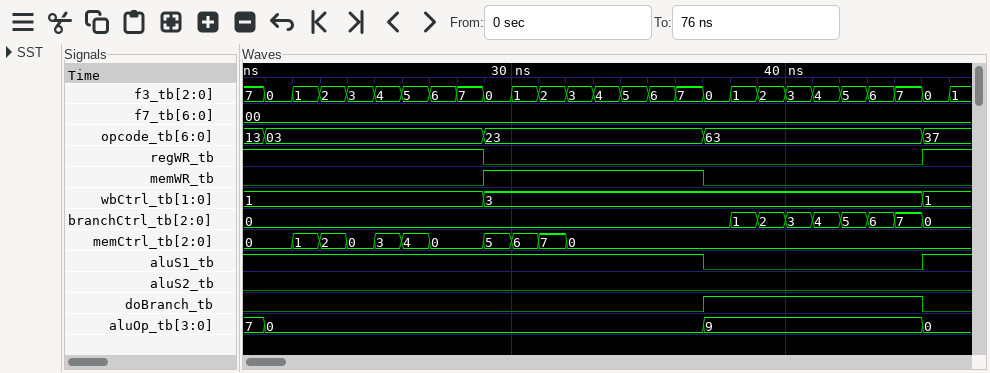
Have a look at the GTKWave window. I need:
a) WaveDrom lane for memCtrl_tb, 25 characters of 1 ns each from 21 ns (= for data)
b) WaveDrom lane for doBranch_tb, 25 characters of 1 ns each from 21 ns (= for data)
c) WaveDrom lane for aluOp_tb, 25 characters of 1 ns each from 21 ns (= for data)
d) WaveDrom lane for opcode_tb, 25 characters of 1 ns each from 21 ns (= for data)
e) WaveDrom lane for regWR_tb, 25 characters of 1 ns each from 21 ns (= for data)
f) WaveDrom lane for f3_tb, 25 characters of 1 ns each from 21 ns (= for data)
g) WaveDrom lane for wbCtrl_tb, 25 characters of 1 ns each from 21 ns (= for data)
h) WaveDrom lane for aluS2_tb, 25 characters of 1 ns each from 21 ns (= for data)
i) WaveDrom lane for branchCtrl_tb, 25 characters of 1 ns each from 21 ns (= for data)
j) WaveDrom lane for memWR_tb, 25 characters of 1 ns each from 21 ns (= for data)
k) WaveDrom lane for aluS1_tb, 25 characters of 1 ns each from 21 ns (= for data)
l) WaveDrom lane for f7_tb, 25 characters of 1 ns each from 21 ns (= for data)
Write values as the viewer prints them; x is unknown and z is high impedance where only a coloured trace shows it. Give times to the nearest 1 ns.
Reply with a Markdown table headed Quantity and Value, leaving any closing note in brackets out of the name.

| Quantity | Value |
|---|---|
| WaveDrom lane for memCtrl_tb, 25 characters of 1 ns each from 21 ns | {name: 'memCtrl_tb', wave: '=======.====.............', data: '0 1 2 0 3 4 0 5 6 7 0'} |
| WaveDrom lane for doBranch_tb, 25 characters of 1 ns each from 21 ns | {name: 'doBranch_tb', wave: '0...............1.......0'} |
| WaveDrom lane for aluOp_tb, 25 characters of 1 ns each from 21 ns | {name: 'aluOp_tb', wave: '=...............=.......=', data: '0 9 0'} |
| WaveDrom lane for opcode_tb, 25 characters of 1 ns each from 21 ns | {name: 'opcode_tb', wave: '=.......=.......=.......=', data: '03 23 63 37'} |
| WaveDrom lane for regWR_tb, 25 characters of 1 ns each from 21 ns | {name: 'regWR_tb', wave: '1.......0...............1'} |
| WaveDrom lane for f3_tb, 25 characters of 1 ns each from 21 ns | {name: 'f3_tb', wave: '=========================', data: '0 1 2 3 4 5 6 7 0 1 2 3 4 5 6 7 0 1 2 3 4 5 6 7 0'} |
| WaveDrom lane for wbCtrl_tb, 25 characters of 1 ns each from 21 ns | {name: 'wbCtrl_tb', wave: '=.......=...............=', data: '1 3 1'} |
| WaveDrom lane for aluS2_tb, 25 characters of 1 ns each from 21 ns | {name: 'aluS2_tb', wave: '0........................'} |
| WaveDrom lane for branchCtrl_tb, 25 characters of 1 ns each from 21 ns | {name: 'branchCtrl_tb', wave: '=................========', data: '0 1 2 3 4 5 6 7 0'} |
| WaveDrom lane for memWR_tb, 25 characters of 1 ns each from 21 ns | {name: 'memWR_tb', wave: '0.......1.......0........'} |
| WaveDrom lane for aluS1_tb, 25 characters of 1 ns each from 21 ns | {name: 'aluS1_tb', wave: '1...............0.......1'} |
| WaveDrom lane for f7_tb, 25 characters of 1 ns each from 21 ns | {name: 'f7_tb', wave: '=........................', data: '00'} |
